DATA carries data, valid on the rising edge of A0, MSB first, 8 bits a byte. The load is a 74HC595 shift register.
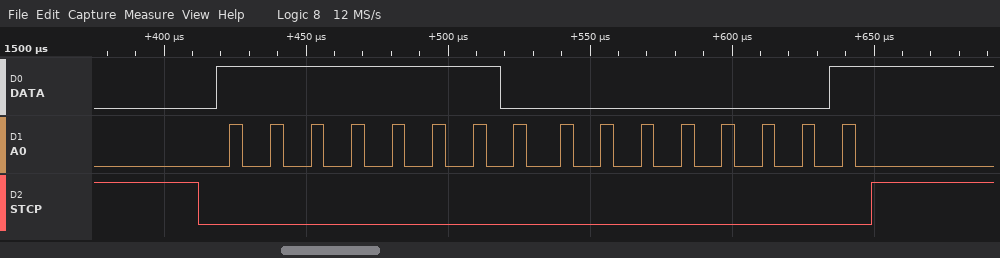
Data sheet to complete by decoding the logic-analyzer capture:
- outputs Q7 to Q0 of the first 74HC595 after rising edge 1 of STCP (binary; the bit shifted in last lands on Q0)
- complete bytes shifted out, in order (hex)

00000001
FE 01
